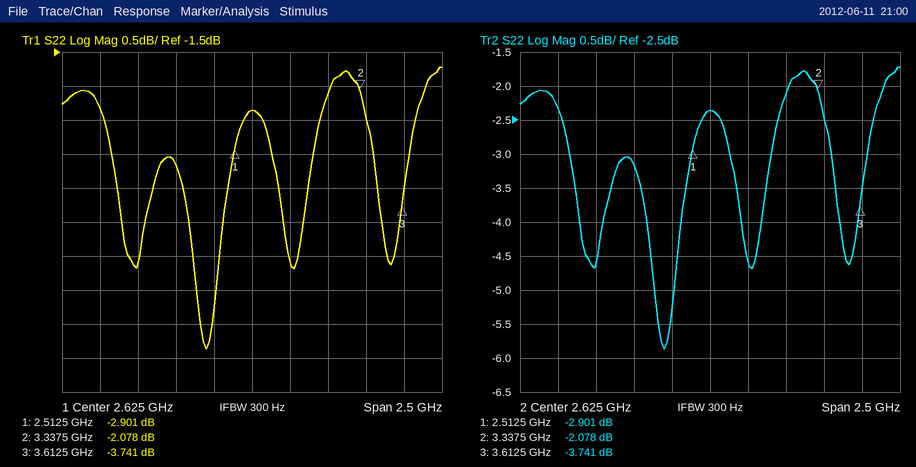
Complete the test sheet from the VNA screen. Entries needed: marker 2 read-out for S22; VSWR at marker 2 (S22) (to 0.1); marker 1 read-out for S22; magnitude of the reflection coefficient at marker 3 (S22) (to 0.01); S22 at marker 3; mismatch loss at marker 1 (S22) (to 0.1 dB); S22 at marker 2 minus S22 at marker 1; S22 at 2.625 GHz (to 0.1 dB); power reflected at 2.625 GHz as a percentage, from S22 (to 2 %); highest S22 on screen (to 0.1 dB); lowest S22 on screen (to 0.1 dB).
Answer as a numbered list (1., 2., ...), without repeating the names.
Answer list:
1. -2.078 dB
2. 8.4
3. -2.901 dB
4. 0.65
5. -3.741 dB
6. 3.1 dB
7. 0.823 dB
8. -2.4 dB
9. 58 %
10. -1.7 dB
11. -5.9 dB
